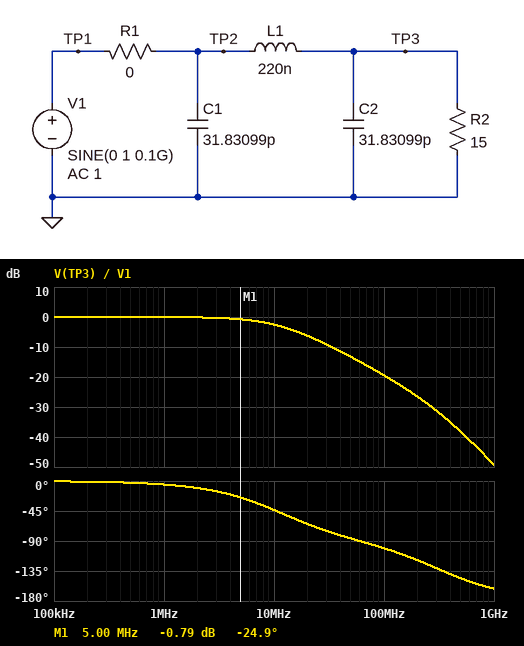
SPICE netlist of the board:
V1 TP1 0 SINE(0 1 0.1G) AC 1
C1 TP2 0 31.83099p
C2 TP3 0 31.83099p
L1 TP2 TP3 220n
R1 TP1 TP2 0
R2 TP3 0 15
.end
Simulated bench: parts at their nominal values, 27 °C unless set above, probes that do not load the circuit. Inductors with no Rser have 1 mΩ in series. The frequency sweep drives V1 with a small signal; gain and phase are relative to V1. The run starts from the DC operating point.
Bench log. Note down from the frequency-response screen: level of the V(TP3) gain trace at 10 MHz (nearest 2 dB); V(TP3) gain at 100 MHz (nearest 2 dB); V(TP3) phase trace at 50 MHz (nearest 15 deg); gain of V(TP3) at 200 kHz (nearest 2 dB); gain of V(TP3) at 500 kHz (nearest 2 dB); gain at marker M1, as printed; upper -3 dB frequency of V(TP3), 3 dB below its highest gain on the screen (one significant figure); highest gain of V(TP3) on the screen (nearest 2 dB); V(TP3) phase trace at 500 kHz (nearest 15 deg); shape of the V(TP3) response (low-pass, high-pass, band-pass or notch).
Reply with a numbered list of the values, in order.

1. -2 dB
2. -20 dB
3. -90 deg
4. 0 dB
5. 0 dB
6. -0.79 dB
7. 10 MHz
8. 0 dB
9. 0 deg
10. low-pass
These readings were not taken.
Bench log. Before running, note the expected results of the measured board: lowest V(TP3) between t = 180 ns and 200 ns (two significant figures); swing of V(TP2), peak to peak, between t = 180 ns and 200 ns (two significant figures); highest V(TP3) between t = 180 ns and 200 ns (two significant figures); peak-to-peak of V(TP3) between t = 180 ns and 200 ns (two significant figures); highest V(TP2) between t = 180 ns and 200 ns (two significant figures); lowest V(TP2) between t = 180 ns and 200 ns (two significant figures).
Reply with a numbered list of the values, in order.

1. -110 mV
2. 2.0 V
3. 110 mV
4. 210 mV
5. 1.0 V
6. -1.0 V
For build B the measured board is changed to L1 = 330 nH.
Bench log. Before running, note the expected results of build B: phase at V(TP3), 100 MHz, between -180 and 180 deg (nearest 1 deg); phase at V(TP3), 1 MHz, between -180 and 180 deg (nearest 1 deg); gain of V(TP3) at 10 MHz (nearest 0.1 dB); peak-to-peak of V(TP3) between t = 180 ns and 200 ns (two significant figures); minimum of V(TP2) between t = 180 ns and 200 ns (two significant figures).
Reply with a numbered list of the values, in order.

1. -103 deg
2. -8 deg
3. -4.5 dB
4. 140 mV
5. -1.0 V
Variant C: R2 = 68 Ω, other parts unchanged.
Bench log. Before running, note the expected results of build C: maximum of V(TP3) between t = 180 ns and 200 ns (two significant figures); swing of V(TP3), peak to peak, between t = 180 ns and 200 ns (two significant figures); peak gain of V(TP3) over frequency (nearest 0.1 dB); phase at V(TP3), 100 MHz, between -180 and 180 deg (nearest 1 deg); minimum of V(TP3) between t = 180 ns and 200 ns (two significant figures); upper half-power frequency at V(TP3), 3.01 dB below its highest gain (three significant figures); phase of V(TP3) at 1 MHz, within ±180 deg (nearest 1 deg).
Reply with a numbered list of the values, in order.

1. 370 mV
2. 740 mV
3. 0.3 dB
4. -131 deg
5. -370 mV
6. 66.4 MHz
7. -1 deg
